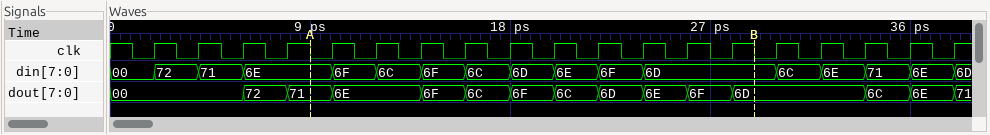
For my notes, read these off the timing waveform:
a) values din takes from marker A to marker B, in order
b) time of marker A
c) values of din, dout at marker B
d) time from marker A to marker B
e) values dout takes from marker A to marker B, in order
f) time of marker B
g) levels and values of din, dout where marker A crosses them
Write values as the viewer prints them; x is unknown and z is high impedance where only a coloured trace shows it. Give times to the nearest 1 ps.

6E, 6F, 6C, 6F, 6C, 6D, 6E, 6F, 6D
9 ps
din=6D, dout=6D
20 ps
71, 6E, 6F, 6C, 6F, 6C, 6D, 6E, 6F, 6D
29 ps
din=6E, dout=71
